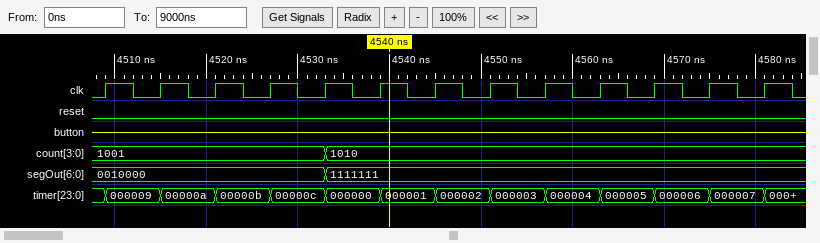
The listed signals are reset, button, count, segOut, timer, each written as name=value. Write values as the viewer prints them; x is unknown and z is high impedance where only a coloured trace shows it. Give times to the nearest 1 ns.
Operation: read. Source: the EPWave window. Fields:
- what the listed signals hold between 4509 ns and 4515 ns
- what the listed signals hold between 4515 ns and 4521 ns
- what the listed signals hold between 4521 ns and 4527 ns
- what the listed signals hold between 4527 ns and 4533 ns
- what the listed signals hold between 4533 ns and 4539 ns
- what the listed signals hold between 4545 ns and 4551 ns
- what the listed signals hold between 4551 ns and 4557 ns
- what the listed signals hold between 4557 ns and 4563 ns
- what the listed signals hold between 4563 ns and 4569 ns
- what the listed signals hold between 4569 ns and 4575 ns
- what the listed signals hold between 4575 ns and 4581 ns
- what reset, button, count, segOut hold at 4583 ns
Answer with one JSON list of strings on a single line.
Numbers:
["reset=0, button=z, count=1001, segOut=0010000, timer=000009", "reset=0, button=z, count=1001, segOut=0010000, timer=00000a", "reset=0, button=z, count=1001, segOut=0010000, timer=00000b", "reset=0, button=z, count=1001, segOut=0010000, timer=00000c", "reset=0, button=z, count=1010, segOut=1111111, timer=000000", "reset=0, button=z, count=1010, segOut=1111111, timer=000002", "reset=0, button=z, count=1010, segOut=1111111, timer=000003", "reset=0, button=z, count=1010, segOut=1111111, timer=000004", "reset=0, button=z, count=1010, segOut=1111111, timer=000005", "reset=0, button=z, count=1010, segOut=1111111, timer=000006", "reset=0, button=z, count=1010, segOut=1111111, timer=000007", "reset=0, button=z, count=1010, segOut=1111111"]
